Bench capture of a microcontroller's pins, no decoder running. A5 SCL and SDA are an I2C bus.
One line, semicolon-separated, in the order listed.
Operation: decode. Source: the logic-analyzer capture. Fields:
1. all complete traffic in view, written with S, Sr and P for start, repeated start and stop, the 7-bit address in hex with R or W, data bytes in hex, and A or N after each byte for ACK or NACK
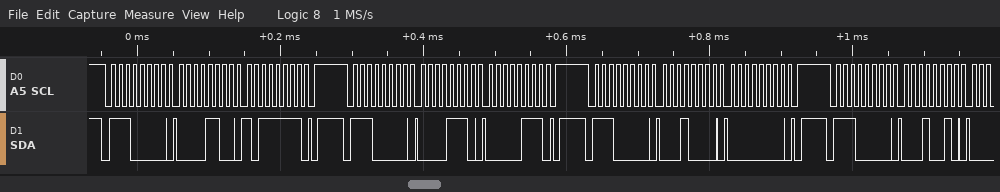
S 70W A 0C A BF A P S 70W A 0E A 07 A P S 70W A 10 A 00 A P S 70W A 12 A
